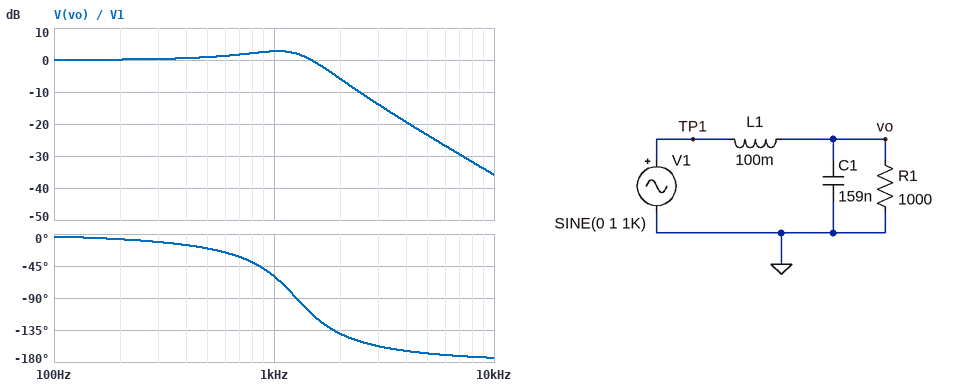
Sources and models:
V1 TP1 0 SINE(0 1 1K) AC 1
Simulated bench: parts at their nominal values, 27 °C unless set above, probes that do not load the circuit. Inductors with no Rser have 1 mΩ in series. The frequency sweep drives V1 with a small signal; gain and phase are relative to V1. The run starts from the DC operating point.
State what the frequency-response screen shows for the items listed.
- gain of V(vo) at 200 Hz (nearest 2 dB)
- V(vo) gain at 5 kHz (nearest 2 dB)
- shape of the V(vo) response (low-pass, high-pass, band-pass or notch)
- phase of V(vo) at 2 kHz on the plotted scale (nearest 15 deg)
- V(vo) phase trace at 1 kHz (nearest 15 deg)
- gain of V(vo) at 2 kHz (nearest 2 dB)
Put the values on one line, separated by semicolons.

0 dB; -24 dB; low-pass; -135 deg; -60 deg; -6 dB
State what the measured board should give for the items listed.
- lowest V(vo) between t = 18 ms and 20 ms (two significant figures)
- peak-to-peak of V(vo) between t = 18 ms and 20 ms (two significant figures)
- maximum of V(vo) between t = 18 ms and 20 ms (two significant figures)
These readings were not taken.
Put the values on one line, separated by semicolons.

-1.4 V; 2.7 V; 1.4 V
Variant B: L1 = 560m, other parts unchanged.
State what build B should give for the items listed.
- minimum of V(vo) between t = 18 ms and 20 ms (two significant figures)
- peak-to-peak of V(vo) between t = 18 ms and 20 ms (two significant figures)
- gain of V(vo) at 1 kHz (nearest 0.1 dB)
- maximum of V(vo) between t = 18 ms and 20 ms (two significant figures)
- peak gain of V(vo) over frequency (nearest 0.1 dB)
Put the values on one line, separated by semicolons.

-230 mV; 460 mV; -12.7 dB; 230 mV; 0 dB
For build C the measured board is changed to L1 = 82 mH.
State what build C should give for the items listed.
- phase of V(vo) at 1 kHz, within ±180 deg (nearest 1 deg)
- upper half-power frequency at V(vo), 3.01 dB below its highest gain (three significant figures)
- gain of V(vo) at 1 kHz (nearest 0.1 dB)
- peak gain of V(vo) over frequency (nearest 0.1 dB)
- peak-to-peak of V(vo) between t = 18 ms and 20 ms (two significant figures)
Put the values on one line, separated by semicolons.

-47 deg; 1.66 kHz; 3.0 dB; 3.5 dB; 2.8 V
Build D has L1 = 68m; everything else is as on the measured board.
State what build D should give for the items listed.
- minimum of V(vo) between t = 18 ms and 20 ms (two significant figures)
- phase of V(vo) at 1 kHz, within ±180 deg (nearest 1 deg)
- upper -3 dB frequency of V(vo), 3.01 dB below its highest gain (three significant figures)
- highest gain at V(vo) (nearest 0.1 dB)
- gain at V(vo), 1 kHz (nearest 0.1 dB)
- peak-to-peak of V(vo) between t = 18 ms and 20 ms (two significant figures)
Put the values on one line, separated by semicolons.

-1.4 V; -37 deg; 1.81 kHz; 4.2 dB; 2.9 dB; 2.8 V
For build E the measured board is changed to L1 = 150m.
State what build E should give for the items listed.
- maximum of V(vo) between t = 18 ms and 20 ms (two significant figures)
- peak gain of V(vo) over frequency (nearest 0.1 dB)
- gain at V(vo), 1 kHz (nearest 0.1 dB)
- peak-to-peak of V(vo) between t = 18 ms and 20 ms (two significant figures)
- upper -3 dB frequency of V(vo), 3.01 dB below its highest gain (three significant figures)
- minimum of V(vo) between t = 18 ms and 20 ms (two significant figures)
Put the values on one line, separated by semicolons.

1.1 V; 1.4 dB; 0.5 dB; 2.1 V; 1.21 kHz; -1.1 V
